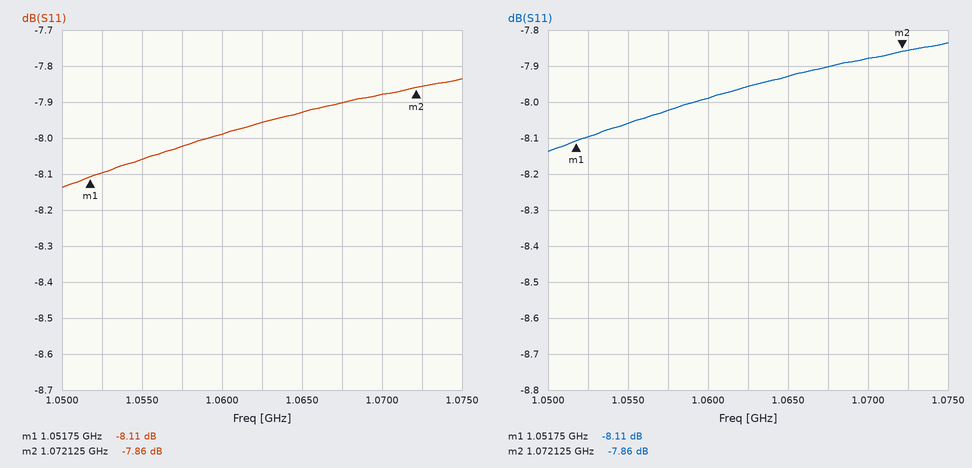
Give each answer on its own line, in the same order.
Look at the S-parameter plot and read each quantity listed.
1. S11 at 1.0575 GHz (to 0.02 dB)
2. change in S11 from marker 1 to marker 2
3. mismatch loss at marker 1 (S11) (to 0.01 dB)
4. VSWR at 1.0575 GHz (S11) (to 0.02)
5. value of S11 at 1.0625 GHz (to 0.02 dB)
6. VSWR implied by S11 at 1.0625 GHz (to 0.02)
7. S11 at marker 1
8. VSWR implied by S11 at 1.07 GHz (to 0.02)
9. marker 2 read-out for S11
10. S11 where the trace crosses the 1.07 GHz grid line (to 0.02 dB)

-8.02 dB
0.25 dB
0.73 dB
2.32
-7.96 dB
2.34
-8.11 dB
2.36
-7.86 dB
-7.88 dB
